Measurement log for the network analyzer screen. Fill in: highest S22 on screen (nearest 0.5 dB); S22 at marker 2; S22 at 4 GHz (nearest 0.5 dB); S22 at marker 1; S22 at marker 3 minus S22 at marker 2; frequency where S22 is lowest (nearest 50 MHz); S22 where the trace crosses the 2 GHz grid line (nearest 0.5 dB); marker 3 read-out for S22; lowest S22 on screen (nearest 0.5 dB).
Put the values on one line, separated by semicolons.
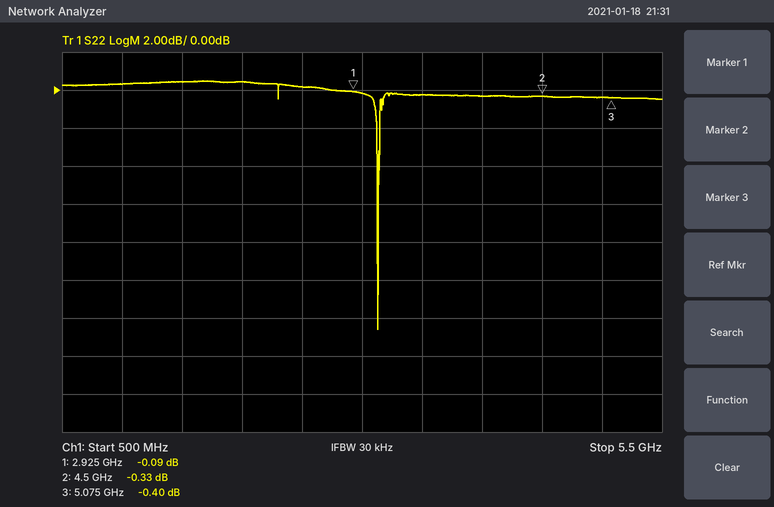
0.5 dB; -0.33 dB; -0.5 dB; -0.09 dB; -0.07 dB; 3.15 GHz; 0.5 dB; -0.40 dB; -12.5 dB
